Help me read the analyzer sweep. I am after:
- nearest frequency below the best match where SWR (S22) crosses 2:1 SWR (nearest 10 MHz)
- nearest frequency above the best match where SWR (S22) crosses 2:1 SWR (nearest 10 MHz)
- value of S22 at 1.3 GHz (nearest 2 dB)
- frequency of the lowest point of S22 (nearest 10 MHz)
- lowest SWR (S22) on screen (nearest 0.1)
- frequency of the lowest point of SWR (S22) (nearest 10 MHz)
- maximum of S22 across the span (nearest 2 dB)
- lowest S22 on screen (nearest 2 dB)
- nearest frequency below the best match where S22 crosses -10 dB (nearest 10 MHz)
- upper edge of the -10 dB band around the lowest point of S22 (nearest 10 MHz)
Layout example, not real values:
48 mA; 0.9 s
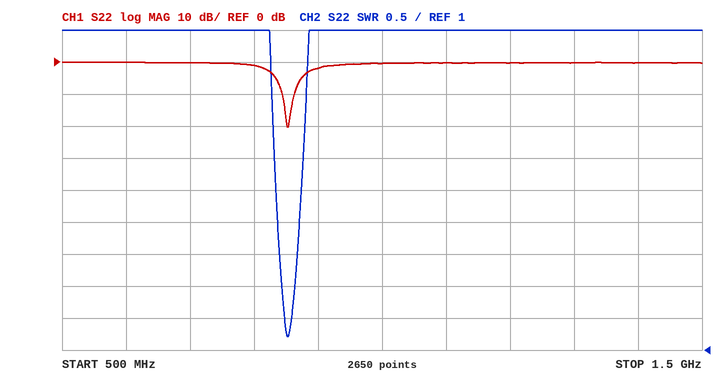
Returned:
840 MHz; 860 MHz; 0 dB; 850 MHz; 1.2; 850 MHz; 0 dB; -20 dB; 840 MHz; 860 MHz
